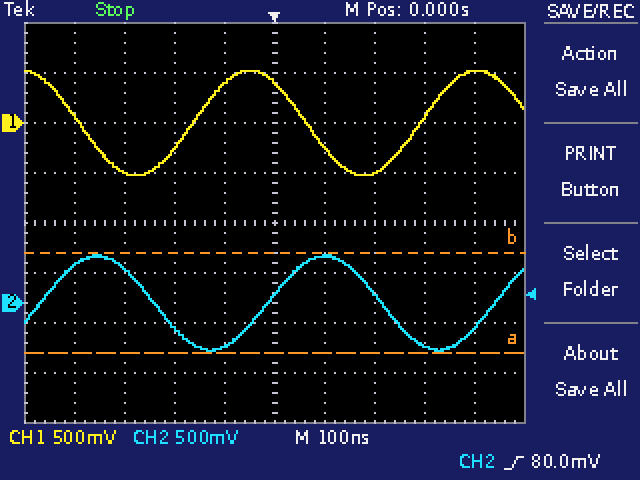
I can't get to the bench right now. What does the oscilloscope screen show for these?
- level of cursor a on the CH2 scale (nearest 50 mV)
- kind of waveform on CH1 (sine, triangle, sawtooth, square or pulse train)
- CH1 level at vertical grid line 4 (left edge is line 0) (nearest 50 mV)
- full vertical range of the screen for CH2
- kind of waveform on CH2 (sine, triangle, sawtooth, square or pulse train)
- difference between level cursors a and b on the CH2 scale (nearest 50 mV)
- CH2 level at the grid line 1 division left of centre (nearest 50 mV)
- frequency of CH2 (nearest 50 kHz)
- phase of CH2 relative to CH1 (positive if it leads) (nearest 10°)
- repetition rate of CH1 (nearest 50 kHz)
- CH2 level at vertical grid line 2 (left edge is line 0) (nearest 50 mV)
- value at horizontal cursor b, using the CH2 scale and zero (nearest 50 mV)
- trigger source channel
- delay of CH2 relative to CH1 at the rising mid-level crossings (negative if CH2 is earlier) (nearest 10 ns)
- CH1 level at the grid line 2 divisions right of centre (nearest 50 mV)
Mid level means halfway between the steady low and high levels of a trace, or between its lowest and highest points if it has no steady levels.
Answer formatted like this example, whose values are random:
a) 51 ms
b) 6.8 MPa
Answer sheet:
a) -500 mV
b) sine
c) 400 mV
d) 4 V
e) sine
f) 1.00 V
g) -450 mV
h) 2.20 MHz
i) -120°
j) 2.20 MHz
k) 350 mV
l) 500 mV
m) CH2
n) +150 ns
o) -500 mV
